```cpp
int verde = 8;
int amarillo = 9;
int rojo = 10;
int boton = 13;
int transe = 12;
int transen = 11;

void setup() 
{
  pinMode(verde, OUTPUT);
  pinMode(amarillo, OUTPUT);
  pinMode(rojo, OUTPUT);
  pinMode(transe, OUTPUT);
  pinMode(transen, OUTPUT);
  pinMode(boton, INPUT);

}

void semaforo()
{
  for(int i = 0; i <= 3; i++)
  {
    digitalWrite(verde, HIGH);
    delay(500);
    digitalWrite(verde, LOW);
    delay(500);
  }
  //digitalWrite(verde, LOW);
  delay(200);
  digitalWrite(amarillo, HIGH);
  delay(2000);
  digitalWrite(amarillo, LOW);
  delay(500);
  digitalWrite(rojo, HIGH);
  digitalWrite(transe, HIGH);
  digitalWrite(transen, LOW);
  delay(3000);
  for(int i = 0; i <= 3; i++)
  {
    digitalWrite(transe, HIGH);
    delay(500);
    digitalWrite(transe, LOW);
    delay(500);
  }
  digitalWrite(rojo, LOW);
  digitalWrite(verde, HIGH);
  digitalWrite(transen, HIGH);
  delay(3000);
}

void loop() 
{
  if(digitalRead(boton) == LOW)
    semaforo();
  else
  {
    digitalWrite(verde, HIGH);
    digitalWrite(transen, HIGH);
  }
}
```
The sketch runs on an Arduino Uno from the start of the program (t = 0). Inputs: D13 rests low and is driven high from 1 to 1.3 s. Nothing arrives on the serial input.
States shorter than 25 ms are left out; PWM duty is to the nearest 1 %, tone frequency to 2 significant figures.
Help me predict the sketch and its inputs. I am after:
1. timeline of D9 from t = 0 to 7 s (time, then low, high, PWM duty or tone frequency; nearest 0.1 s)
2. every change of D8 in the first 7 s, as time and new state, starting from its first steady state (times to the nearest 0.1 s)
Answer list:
0 s low; 4.2 s high; 6.2 s low
0 s high; 0.5 s low; 1 s high; 1.5 s low; 2 s high; 2.5 s low; 3 s high; 3.5 s low
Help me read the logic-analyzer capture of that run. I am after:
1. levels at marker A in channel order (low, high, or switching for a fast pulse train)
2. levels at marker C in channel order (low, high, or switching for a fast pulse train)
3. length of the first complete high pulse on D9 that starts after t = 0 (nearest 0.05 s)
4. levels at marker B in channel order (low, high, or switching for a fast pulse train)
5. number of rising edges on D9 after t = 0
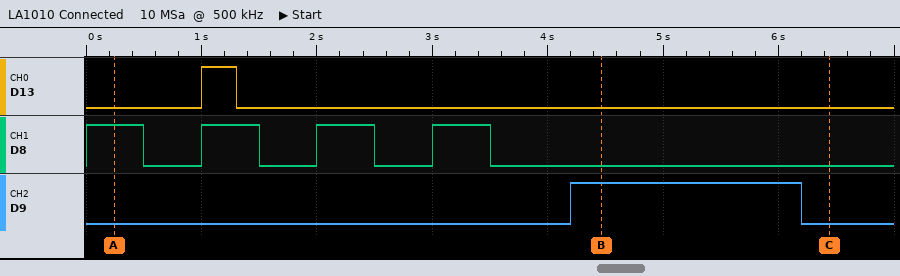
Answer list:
D13 low, D8 high, D9 low
D13 low, D8 low, D9 low
2.00 s
D13 low, D8 low, D9 high
1
